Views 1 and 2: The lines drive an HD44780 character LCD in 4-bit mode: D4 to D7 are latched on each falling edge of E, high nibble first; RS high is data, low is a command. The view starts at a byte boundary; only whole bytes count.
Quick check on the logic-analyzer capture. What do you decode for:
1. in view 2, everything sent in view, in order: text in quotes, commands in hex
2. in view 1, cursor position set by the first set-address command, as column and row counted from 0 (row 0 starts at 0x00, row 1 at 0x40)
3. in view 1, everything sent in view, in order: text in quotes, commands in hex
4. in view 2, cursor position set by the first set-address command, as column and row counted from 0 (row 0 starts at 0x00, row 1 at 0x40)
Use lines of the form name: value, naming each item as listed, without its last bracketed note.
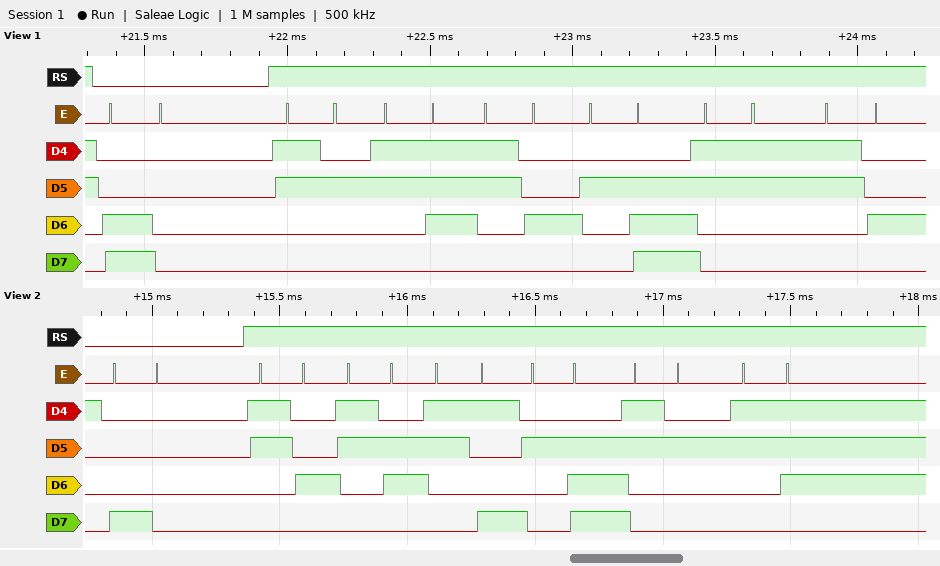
in view 2, everything sent in view, in order: text in quotes, commands in hex: 0x80 "469.27"
in view 1, cursor position set by the first set-address command, as column and row counted from 0: column 0, row 1
in view 1, everything sent in view, in order: text in quotes, commands in hex: 0xC0 "274.34"
in view 2, cursor position set by the first set-address command, as column and row counted from 0: column 0, row 0
